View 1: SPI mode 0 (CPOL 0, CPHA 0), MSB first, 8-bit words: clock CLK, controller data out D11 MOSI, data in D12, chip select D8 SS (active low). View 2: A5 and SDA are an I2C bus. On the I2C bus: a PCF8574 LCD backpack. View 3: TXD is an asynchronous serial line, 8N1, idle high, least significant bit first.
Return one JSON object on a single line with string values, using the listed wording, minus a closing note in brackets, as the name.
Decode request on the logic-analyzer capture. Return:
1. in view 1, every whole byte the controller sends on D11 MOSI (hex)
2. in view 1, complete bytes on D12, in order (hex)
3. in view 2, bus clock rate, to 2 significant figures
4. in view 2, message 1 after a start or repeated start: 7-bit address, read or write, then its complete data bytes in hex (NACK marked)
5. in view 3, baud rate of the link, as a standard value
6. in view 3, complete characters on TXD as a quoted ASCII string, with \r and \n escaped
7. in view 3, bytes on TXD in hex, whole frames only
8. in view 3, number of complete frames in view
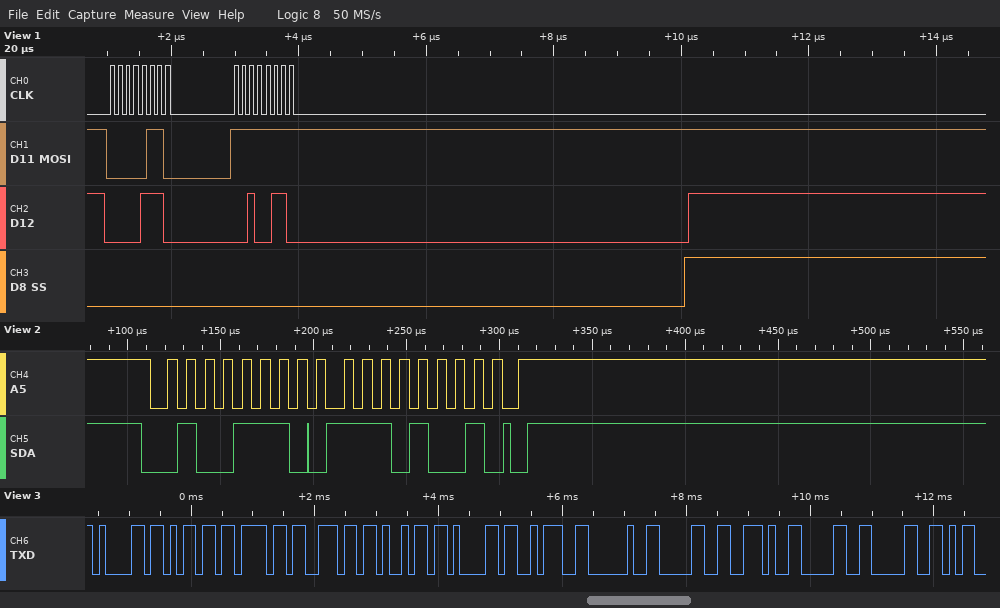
{"in view 1, every whole byte the controller sends on D11 MOSI": "06 FF", "in view 1, complete bytes on D12, in order": "0E 26", "in view 2, bus clock rate, to 2 significant figures": "100 kHz", "in view 2, message 1 after a start or repeated start: 7-bit address, read or write, then its complete data bytes in hex": "0x27 write: E9", "in view 3, baud rate of the link, as a standard value": "9600 baud", "in view 3, complete characters on TXD as a quoted ASCII string, with \\r and \\n escaped": "\"amonia: 0.00\"", "in view 3, bytes on TXD in hex, whole frames only": "0x61 0x6D 0x6F 0x6E 0x69 0x61 0x3A 0x20 0x30 0x2E 0x30 0x30", "in view 3, number of complete frames in view": "12"}
